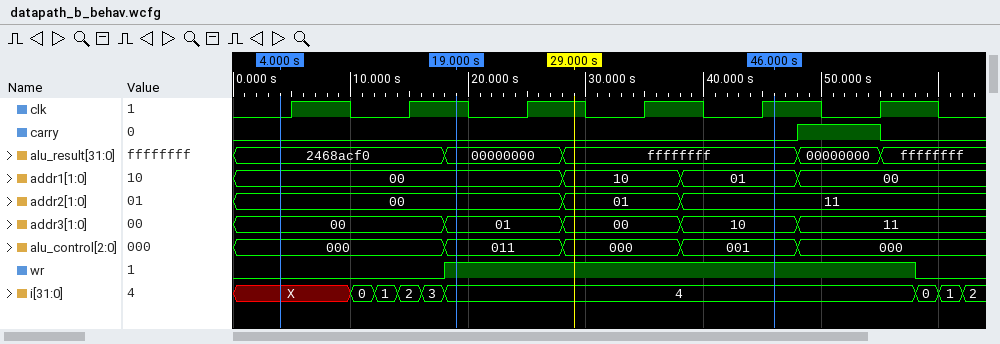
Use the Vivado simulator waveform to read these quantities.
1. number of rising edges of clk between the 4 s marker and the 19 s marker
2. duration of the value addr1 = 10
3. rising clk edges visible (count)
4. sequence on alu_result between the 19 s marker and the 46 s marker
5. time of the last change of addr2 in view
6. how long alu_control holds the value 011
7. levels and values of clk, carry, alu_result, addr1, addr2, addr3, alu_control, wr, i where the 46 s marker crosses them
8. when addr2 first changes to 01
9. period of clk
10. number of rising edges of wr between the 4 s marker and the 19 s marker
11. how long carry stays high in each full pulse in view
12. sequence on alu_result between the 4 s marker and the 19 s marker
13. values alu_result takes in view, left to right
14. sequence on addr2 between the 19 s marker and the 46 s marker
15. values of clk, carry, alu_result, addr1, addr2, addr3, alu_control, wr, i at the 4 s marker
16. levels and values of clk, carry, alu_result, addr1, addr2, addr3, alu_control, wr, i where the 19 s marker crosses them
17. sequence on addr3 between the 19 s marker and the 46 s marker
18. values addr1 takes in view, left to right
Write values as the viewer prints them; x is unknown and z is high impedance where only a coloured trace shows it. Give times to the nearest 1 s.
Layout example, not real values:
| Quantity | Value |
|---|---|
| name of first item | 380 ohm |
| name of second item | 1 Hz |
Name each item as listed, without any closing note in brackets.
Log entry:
| Quantity | Value |
|---|---|
| number of rising edges of clk between the 4 s marker and the 19 s marker | 2 |
| duration of the value addr1 = 10 | 10 s |
| rising clk edges visible | 6 |
| sequence on alu_result between the 19 s marker and the 46 s marker | 00000000, ffffffff |
| time of the last change of addr2 in view | 38 s |
| how long alu_control holds the value 011 | 10 s |
| levels and values of clk, carry, alu_result, addr1, addr2, addr3, alu_control, wr, i where the 46 s marker crosses them | clk=1, carry=0, alu_result=ffffffff, addr1=01, addr2=11, addr3=10, alu_control=001, wr=1, i=4 |
| when addr2 first changes to 01 | 28 s |
| period of clk | 10 s |
| number of rising edges of wr between the 4 s marker and the 19 s marker | 1 |
| how long carry stays high in each full pulse in view | 7 s |
| sequence on alu_result between the 4 s marker and the 19 s marker | 2468acf0, 00000000 |
| values alu_result takes in view, left to right | 2468acf0, 00000000, ffffffff, 00000000, ffffffff |
| sequence on addr2 between the 19 s marker and the 46 s marker | 00, 01, 11 |
| values of clk, carry, alu_result, addr1, addr2, addr3, alu_control, wr, i at the 4 s marker | clk=0, carry=0, alu_result=2468acf0, addr1=00, addr2=00, addr3=00, alu_control=000, wr=0, i=X |
| levels and values of clk, carry, alu_result, addr1, addr2, addr3, alu_control, wr, i where the 19 s marker crosses them | clk=1, carry=0, alu_result=00000000, addr1=00, addr2=00, addr3=01, alu_control=011, wr=1, i=4 |
| sequence on addr3 between the 19 s marker and the 46 s marker | 01, 00, 10 |
| values addr1 takes in view, left to right | 00, 10, 01, 00 |
